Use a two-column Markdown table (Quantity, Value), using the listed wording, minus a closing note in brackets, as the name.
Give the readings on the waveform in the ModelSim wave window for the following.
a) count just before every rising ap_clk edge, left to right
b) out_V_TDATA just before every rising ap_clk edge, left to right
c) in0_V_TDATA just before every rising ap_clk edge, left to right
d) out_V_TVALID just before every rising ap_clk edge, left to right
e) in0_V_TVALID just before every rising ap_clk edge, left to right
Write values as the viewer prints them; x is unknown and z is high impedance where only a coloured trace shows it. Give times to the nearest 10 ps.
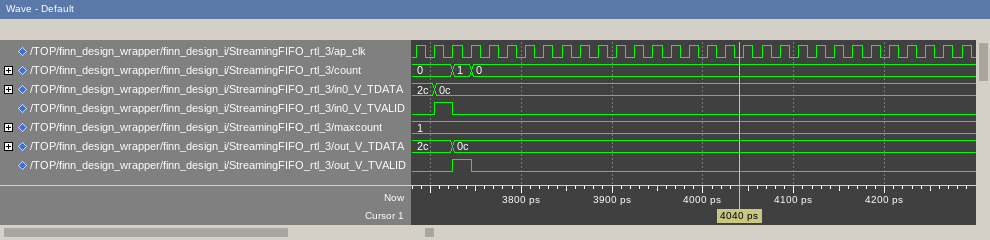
| Quantity | Value |
|---|---|
| count just before every rising ap_clk edge, left to right | 0, 0, 0, 1, 0, 0, 0, 0, 0, 0, 0, 0, 0, 0, 0, 0, 0, 0, 0, 0, 0, 0, 0, 0, 0, 0, 0, 0, 0, 0, 0 |
| out_V_TDATA just before every rising ap_clk edge, left to right | 2c, 2c, 2c, 0c, 0c, 0c, 0c, 0c, 0c, 0c, 0c, 0c, 0c, 0c, 0c, 0c, 0c, 0c, 0c, 0c, 0c, 0c, 0c, 0c, 0c, 0c, 0c, 0c, 0c, 0c, 0c |
| in0_V_TDATA just before every rising ap_clk edge, left to right | 2c, 2c, 0c, 0c, 0c, 0c, 0c, 0c, 0c, 0c, 0c, 0c, 0c, 0c, 0c, 0c, 0c, 0c, 0c, 0c, 0c, 0c, 0c, 0c, 0c, 0c, 0c, 0c, 0c, 0c, 0c |
| out_V_TVALID just before every rising ap_clk edge, left to right | 0 0 0 1 0 0 0 0 0 0 0 0 0 0 0 0 0 0 0 0 0 0 0 0 0 0 0 0 0 0 0 |
| in0_V_TVALID just before every rising ap_clk edge, left to right | 0 0 1 0 0 0 0 0 0 0 0 0 0 0 0 0 0 0 0 0 0 0 0 0 0 0 0 0 0 0 0 |
